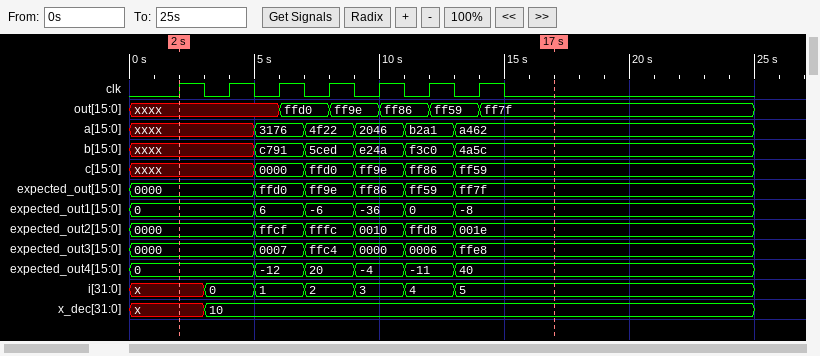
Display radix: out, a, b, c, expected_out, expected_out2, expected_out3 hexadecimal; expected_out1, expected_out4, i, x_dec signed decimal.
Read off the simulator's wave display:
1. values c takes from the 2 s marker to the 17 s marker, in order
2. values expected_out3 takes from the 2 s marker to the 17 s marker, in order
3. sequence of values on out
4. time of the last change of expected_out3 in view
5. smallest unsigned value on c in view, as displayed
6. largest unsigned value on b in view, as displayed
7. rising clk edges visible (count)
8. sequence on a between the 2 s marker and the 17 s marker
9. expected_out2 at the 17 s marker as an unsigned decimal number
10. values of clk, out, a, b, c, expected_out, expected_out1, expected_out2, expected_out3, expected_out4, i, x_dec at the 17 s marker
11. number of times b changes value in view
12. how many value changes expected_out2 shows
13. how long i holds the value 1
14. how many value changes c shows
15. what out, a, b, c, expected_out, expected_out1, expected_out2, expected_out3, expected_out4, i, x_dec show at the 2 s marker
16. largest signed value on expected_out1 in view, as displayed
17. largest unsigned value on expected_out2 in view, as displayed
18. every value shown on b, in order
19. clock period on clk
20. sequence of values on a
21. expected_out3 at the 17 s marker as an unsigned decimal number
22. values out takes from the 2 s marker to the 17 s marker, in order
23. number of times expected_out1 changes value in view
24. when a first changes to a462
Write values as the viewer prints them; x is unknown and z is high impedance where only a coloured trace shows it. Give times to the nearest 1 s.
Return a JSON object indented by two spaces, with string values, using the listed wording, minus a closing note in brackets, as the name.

{
  "values c takes from the 2 s marker to the 17 s marker, in order": "xxxx, 0000, ffd0, ff9e, ff86, ff59",
  "values expected_out3 takes from the 2 s marker to the 17 s marker, in order": "0000, 0007, ffc4, 0000, 0006, ffe8",
  "sequence of values on out": "xxxx, ffd0, ff9e, ff86, ff59, ff7f",
  "time of the last change of expected_out3 in view": "13 s",
  "smallest unsigned value on c in view, as displayed": "0000",
  "largest unsigned value on b in view, as displayed": "f3c0",
  "rising clk edges visible": "7",
  "sequence on a between the 2 s marker and the 17 s marker": "xxxx, 3176, 4f22, 2046, b2a1, a462",
  "expected_out2 at the 17 s marker as an unsigned decimal number": "30",
  "values of clk, out, a, b, c, expected_out, expected_out1, expected_out2, expected_out3, expected_out4, i, x_dec at the 17 s marker": "clk=0, out=ff7f, a=a462, b=4a5c, c=ff59, expected_out=ff7f, expected_out1=-8, expected_out2=001e, expected_out3=ffe8, expected_out4=40, i=5, x_dec=10",
  "number of times b changes value in view": "5",
  "how many value changes expected_out2 shows": "5",
  "how long i holds the value 1": "2 s",
  "how many value changes c shows": "5",
  "what out, a, b, c, expected_out, expected_out1, expected_out2, expected_out3, expected_out4, i, x_dec show at the 2 s marker": "out=xxxx, a=xxxx, b=xxxx, c=xxxx, expected_out=0000, expected_out1=0, expected_out2=0000, expected_out3=0000, expected_out4=0, i=x, x_dec=x",
  "largest signed value on expected_out1 in view, as displayed": "6",
  "largest unsigned value on expected_out2 in view, as displayed": "fffc",
  "every value shown on b, in order": "xxxx, c791, 5ced, e24a, f3c0, 4a5c",
  "clock period on clk": "2 s",
  "sequence of values on a": "xxxx, 3176, 4f22, 2046, b2a1, a462",
  "expected_out3 at the 17 s marker as an unsigned decimal number": "65512",
  "values out takes from the 2 s marker to the 17 s marker, in order": "xxxx, ffd0, ff9e, ff86, ff59, ff7f",
  "number of times expected_out1 changes value in view": "5",
  "when a first changes to a462": "13 s"
}
